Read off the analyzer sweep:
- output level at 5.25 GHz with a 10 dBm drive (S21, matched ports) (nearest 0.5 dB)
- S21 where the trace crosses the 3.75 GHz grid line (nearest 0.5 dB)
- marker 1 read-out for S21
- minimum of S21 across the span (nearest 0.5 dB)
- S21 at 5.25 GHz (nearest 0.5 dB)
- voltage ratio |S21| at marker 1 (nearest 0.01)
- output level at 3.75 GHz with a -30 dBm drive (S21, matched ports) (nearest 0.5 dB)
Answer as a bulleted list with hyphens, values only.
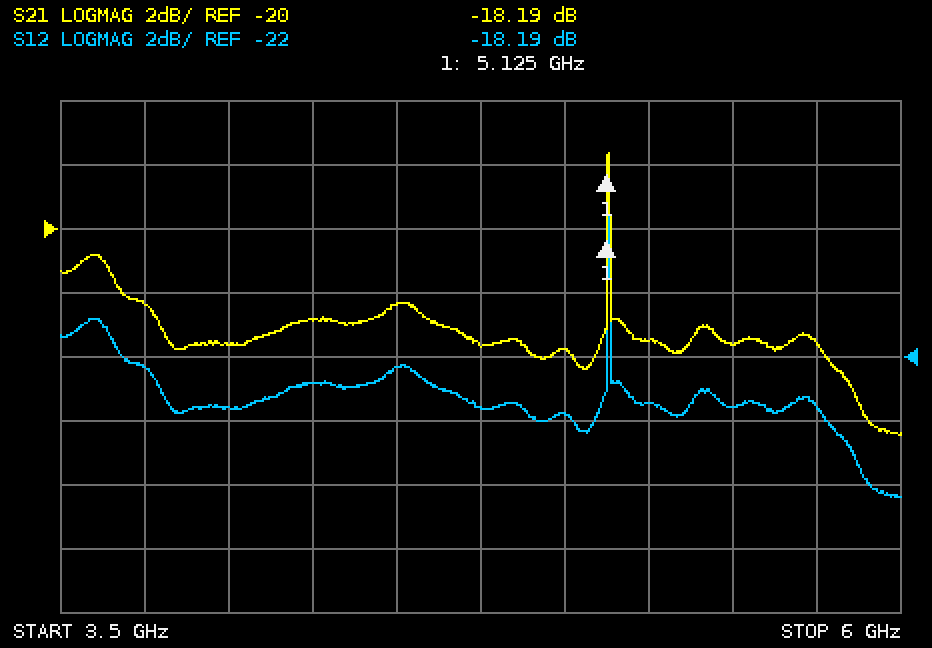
- -13.5 dBm
- -22.5 dB
- -18.19 dB
- -26.5 dB
- -23.5 dB
- 0.12
- -52.5 dBm
